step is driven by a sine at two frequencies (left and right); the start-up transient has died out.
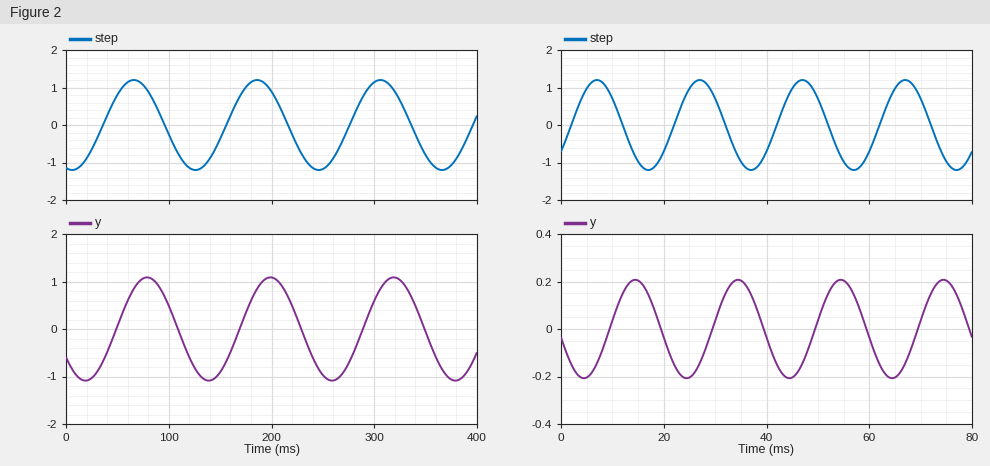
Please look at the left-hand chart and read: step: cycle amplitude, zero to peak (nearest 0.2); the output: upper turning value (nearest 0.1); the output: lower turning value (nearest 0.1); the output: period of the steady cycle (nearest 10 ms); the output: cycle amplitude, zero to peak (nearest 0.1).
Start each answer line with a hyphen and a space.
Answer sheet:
- 1.2
- 1.1
- -1.1
- 120 ms
- 1.1
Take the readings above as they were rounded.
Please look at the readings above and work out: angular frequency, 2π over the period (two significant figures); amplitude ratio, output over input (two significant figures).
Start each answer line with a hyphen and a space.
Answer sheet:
- 0.052 rad/ms
- 0.92
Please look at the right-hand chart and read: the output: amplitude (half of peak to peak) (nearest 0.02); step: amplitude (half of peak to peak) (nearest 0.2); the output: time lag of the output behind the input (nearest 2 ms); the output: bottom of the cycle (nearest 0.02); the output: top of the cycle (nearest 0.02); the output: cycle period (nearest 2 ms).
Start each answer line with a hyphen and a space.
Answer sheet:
- 0.20
- 1.2
- 8 ms
- -0.20
- 0.20
- 20 ms
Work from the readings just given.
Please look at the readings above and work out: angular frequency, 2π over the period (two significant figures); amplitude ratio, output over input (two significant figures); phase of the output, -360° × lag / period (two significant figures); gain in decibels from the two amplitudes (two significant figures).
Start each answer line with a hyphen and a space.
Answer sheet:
- 0.31 rad/ms
- 0.17
- -140°
- -16 dB
